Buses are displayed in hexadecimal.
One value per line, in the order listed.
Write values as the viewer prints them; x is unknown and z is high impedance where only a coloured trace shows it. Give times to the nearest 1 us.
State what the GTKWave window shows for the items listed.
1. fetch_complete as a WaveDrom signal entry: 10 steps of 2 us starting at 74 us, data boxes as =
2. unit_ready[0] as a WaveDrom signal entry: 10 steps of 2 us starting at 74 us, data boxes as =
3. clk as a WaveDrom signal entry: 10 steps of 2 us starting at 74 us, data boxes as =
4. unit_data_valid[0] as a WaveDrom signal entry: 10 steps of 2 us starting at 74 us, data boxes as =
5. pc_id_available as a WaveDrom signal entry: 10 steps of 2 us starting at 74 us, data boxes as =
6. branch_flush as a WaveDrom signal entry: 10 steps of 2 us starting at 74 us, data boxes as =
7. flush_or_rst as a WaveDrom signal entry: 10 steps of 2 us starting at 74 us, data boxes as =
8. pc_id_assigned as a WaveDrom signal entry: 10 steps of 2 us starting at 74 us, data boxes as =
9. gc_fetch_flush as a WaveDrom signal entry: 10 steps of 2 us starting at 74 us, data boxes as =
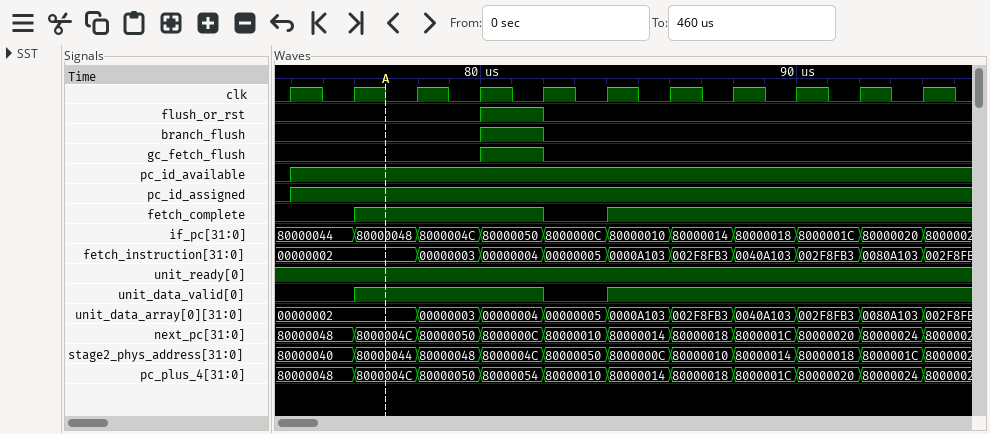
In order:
{name: 'fetch_complete', wave: '01..01....'}
{name: 'unit_ready[0]', wave: '1.........'}
{name: 'clk', wave: 'p.........'}
{name: 'unit_data_valid[0]', wave: '01..01....'}
{name: 'pc_id_available', wave: '1.........'}
{name: 'branch_flush', wave: '0..10.....'}
{name: 'flush_or_rst', wave: '0..10.....'}
{name: 'pc_id_assigned', wave: '1.........'}
{name: 'gc_fetch_flush', wave: '0..10.....'}
